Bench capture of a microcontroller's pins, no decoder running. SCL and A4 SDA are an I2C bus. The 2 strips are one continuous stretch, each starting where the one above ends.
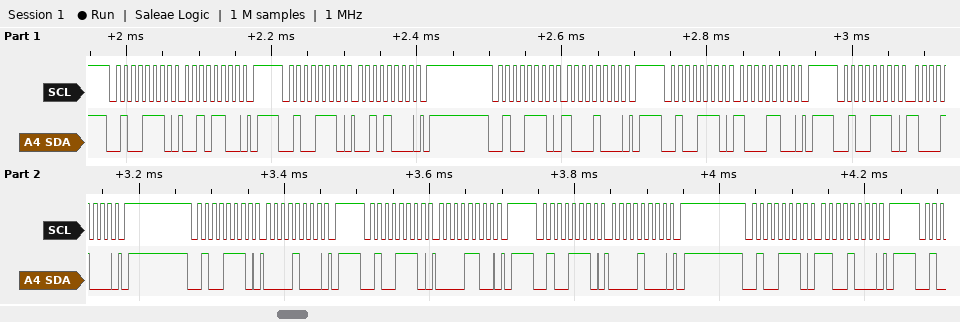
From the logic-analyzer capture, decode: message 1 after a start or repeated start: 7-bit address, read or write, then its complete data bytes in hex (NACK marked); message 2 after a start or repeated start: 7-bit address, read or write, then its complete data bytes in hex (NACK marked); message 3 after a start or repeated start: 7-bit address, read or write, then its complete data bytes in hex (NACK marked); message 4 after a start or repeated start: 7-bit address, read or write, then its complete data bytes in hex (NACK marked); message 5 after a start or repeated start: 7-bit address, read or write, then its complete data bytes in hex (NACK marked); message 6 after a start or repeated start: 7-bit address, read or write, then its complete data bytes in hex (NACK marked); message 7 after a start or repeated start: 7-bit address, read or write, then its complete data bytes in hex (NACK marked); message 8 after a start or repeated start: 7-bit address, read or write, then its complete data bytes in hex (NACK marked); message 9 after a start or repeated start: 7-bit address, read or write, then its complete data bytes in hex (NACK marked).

0x27 write: 2C
0x27 write: 28
0x27 write: 88
0x27 write: 8C
0x27 write: 88
0x27 write: 08
0x27 write: 0C
0x27 write: 08
0x27 write: C8
